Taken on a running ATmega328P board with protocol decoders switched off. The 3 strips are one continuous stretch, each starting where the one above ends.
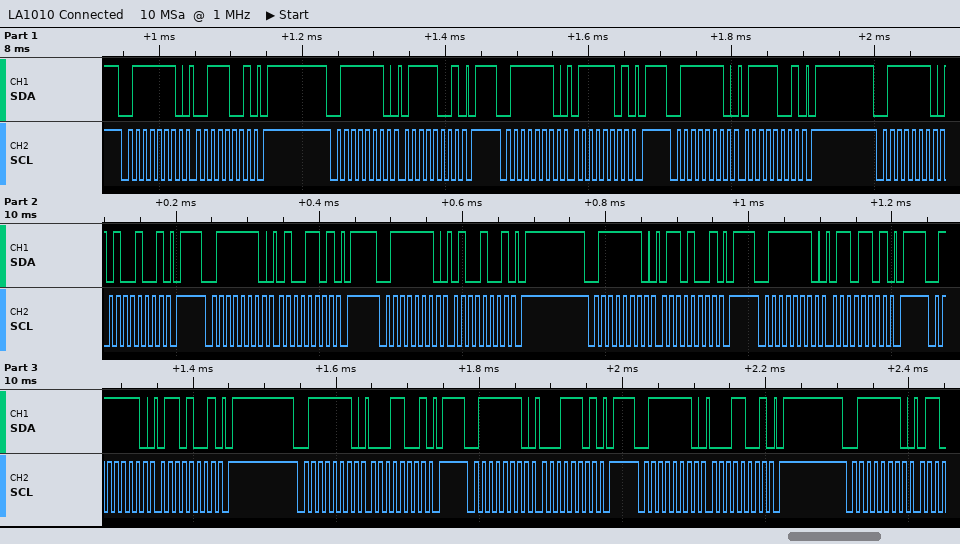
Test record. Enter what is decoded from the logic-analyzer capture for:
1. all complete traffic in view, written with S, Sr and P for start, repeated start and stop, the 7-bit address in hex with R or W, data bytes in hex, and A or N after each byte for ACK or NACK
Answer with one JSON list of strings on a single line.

["S 3FW A 39 A P S 3FW A 79 A P S 3FW A 7D A P S 3FW A 79 A P S 3FW A 49 A P S 3FW A 4D A P S 3FW A 49 A P S 3FW A 69 A P S 3FW A 6D A P S 3FW A 69 A P S 3FW A 19 A P S 3FW A 1D A P S 3FW A 19 A P S 3FW A"]
